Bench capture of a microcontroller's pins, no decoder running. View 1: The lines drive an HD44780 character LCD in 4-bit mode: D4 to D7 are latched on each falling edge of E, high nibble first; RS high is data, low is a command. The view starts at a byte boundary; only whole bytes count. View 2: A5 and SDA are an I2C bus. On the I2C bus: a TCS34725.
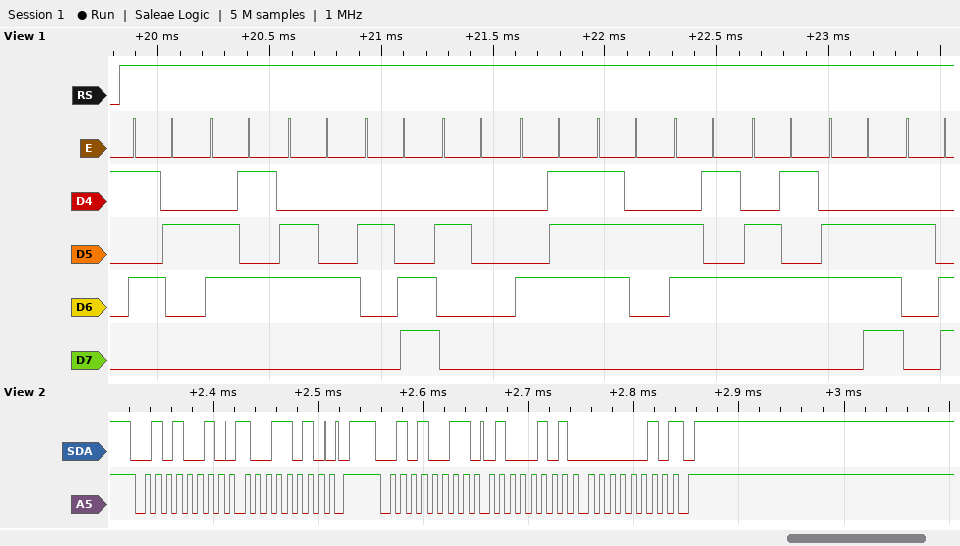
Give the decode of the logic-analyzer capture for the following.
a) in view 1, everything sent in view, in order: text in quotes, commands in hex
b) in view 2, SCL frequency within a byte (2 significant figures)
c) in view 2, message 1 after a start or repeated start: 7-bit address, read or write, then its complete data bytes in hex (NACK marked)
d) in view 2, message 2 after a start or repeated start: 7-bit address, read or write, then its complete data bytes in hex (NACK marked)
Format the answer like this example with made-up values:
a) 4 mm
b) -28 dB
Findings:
a) "Red, Green,"
b) 100 kHz
c) 0x29 write: 9A
d) 0x29 read: 45 02 NACK
